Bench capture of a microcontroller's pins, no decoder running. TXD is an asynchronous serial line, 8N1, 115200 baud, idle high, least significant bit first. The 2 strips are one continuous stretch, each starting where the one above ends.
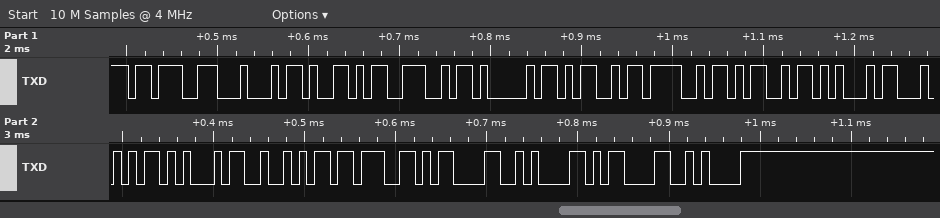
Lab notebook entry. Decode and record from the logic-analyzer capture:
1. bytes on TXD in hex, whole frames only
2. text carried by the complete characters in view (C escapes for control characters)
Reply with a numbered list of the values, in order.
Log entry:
1. 0x3B 0x44 0x59 0x4E 0x41 0x4D 0x4F 0x4D 0x45 0x54 0x45 0x52 0x3B 0x0D 0x0A 0x0D 0x0A
2. ";DYNAMOMETER;\r\n\r\n"
